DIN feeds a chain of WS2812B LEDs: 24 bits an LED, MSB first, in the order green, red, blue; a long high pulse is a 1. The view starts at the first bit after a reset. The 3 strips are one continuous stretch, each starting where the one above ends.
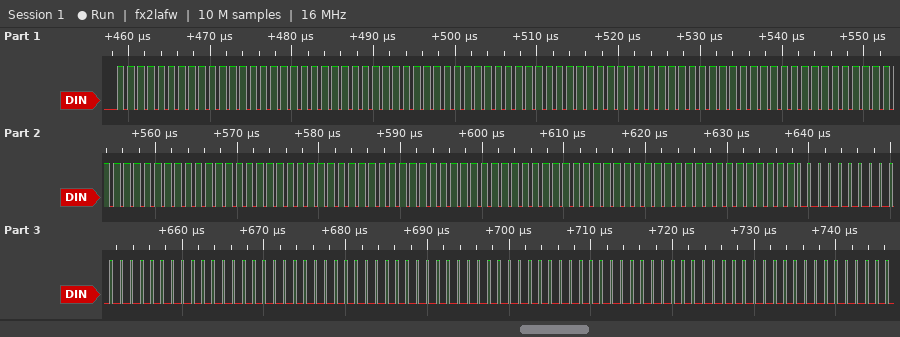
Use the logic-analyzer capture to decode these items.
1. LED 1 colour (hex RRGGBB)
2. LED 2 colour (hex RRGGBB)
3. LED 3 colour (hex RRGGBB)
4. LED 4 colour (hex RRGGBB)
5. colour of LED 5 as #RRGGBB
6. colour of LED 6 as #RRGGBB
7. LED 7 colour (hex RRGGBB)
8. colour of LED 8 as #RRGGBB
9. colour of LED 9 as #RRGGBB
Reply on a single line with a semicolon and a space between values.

#FFFFFF; #FFFFFF; #FFFFFF; #FFFFFF; #FFFFFF; #FFFFFF; #000000; #000000; #000000
